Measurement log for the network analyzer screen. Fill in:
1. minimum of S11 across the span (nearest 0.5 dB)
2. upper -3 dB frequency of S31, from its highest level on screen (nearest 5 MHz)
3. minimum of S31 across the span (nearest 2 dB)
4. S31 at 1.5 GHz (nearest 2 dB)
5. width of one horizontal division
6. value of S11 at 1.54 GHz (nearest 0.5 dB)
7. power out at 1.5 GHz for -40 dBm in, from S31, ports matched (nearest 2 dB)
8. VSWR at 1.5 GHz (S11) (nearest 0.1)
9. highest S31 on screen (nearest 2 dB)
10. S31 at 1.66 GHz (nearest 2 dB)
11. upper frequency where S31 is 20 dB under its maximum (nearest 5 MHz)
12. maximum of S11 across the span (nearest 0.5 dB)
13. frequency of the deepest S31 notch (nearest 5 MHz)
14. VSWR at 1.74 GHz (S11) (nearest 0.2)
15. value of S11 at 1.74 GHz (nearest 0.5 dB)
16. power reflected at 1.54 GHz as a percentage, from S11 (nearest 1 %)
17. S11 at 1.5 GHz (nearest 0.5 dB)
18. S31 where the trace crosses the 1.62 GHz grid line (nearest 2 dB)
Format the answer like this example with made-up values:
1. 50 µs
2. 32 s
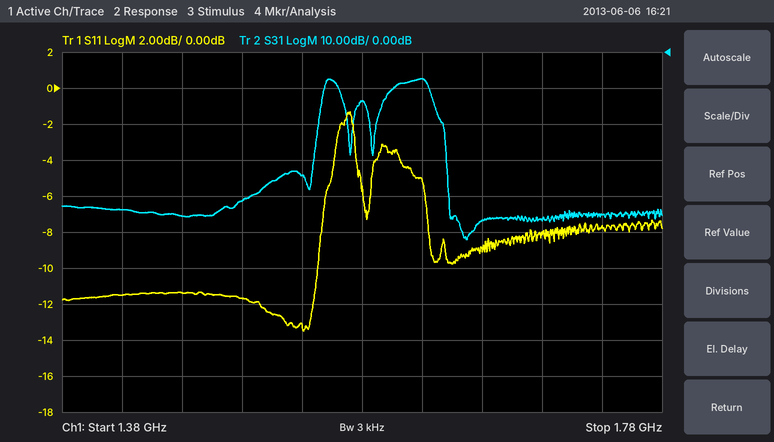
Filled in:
1. -13.5 dB
2. 1.625 GHz
3. -52 dB
4. -42 dB
5. 40 MHz
6. -13.0 dB
7. -82 dBm
8. 1.7
9. -8 dB
10. -46 dB
11. 1.635 GHz
12. -1.5 dB
13. 1.650 GHz
14. 2.4
15. -7.5 dB
16. 5 %
17. -11.5 dB
18. -8 dB
